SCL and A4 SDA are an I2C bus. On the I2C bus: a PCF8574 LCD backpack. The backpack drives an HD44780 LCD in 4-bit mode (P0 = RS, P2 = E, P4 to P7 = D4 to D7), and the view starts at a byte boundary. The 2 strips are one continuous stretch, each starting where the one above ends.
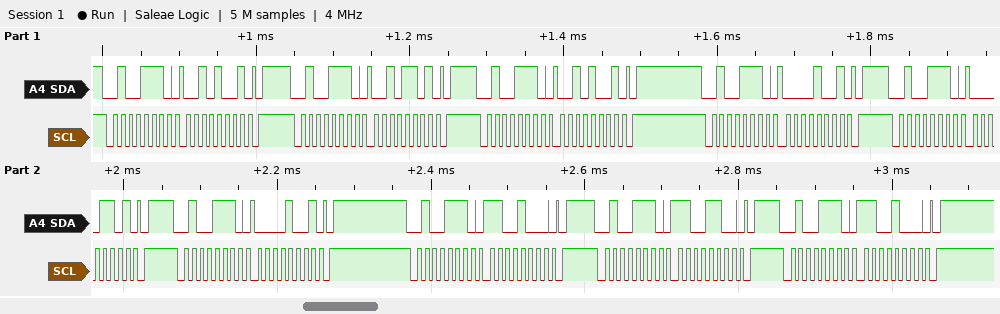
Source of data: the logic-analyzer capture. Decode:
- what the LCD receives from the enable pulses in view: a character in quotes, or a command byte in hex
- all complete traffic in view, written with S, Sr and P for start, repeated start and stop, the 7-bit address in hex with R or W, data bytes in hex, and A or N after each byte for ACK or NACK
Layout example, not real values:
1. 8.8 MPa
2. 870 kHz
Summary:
1. ' '
2. S 27W A 29 A P S 27W A 2D A P S 27W A 29 A P S 27W A 09 A P S 27W A 0D A P S 27W A 09 A P S 27W A C8 A P S 27W A CC A P S 27W A C8 A P
